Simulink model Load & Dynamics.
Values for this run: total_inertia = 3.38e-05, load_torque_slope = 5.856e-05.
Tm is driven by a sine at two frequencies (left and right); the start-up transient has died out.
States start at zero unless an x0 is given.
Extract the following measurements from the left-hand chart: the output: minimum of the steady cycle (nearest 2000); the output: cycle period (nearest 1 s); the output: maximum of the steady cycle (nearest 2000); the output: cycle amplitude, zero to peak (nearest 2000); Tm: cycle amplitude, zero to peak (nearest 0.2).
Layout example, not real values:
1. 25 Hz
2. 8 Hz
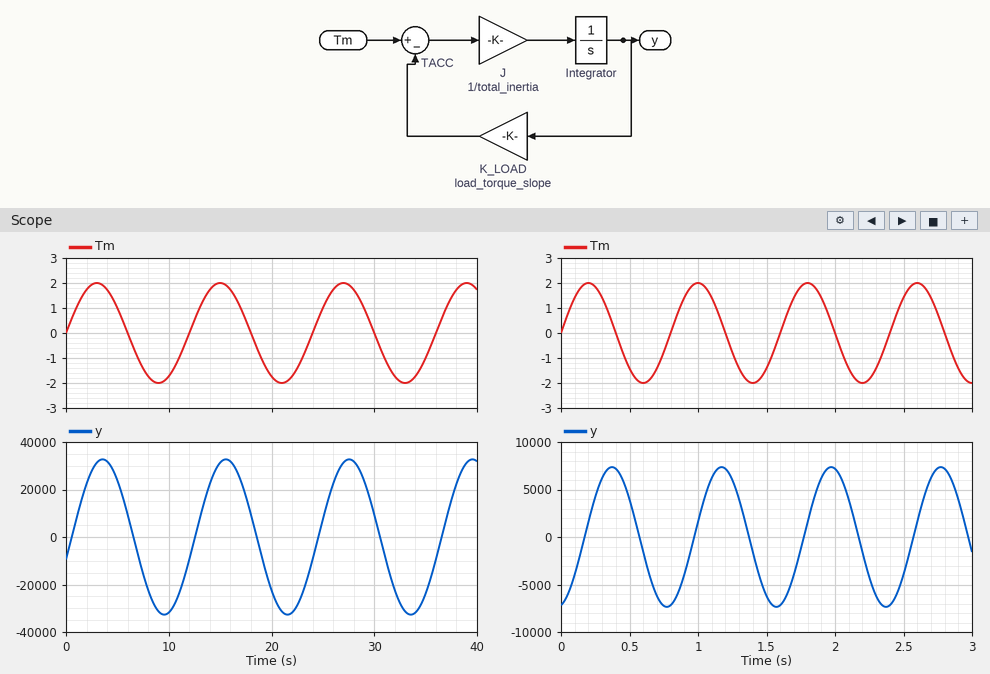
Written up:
1. -32000
2. 12 s
3. 32000
4. 32000
5. 2.0
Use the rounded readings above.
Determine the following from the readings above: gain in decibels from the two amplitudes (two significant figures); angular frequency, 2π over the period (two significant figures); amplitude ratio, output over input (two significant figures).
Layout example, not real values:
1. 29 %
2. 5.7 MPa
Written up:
1. 84 dB
2. 0.52 rad/s
3. 16000
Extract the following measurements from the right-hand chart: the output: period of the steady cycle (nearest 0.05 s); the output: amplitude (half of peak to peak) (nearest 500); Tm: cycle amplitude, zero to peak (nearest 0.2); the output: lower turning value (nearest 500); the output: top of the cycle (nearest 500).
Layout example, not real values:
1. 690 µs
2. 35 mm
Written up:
1. 0.80 s
2. 7500
3. 2.0
4. -7500
5. 7500
